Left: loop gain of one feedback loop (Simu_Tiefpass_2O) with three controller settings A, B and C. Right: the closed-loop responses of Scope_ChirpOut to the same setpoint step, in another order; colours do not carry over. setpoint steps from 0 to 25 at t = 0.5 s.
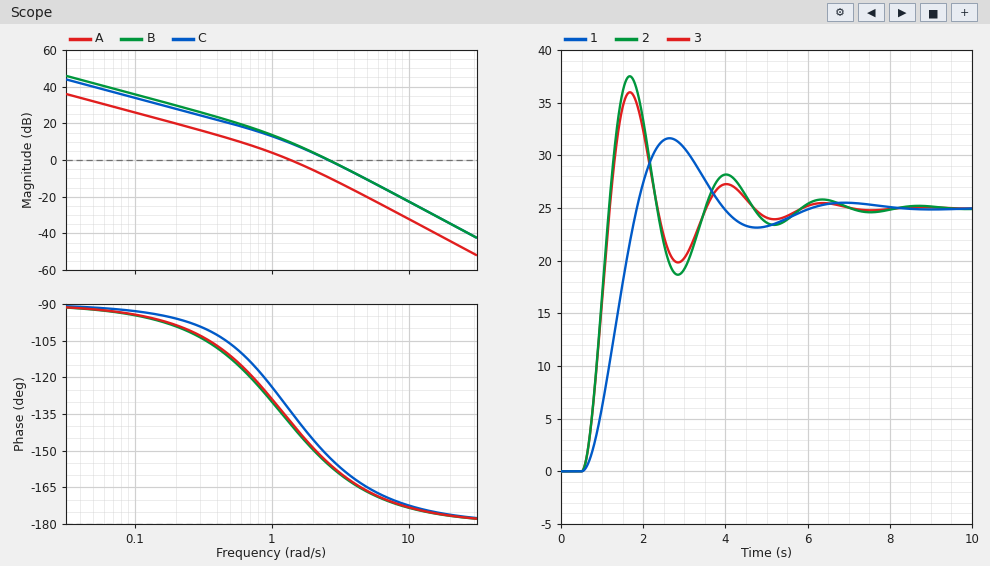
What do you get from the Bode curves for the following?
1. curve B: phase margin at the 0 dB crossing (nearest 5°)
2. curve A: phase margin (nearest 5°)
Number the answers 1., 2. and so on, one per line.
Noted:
1. 25°
2. 40°
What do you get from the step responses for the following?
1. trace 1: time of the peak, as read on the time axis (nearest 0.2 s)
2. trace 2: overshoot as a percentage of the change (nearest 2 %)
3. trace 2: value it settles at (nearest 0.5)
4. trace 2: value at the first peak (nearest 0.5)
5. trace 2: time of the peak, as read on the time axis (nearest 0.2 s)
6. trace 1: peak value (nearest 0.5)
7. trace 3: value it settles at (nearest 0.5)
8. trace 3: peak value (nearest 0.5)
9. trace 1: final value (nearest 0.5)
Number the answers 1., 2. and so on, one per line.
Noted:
1. 2.6 s
2. 50 %
3. 25.0
4. 37.5
5. 1.6 s
6. 31.5
7. 25.0
8. 36.0
9. 25.0
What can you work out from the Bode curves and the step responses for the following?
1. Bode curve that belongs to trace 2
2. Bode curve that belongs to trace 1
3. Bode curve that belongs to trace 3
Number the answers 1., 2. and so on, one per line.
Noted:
1. B
2. A
3. C
